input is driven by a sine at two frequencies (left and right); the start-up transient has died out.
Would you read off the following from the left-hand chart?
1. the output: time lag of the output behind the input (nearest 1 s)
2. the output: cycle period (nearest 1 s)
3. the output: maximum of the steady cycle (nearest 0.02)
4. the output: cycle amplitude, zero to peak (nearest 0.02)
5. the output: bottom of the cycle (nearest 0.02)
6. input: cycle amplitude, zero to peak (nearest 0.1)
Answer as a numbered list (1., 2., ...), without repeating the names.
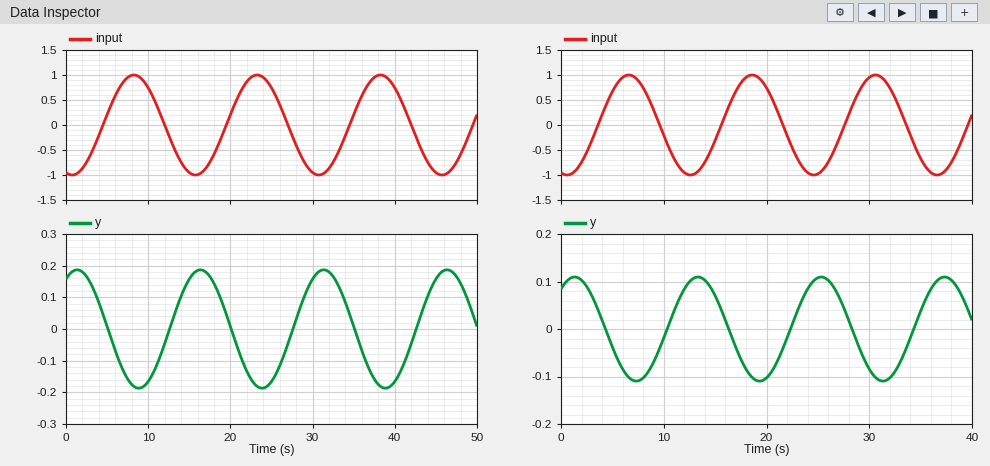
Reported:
1. 8 s
2. 15 s
3. 0.18
4. 0.18
5. -0.18
6. 1.0
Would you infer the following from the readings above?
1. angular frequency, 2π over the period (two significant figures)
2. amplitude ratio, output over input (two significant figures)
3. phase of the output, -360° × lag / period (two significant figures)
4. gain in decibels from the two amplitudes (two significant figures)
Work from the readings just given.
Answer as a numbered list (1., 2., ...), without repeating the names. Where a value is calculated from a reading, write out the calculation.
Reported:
1. 2π / 15 = 0.42 rad/s
2. 0.18 / 1 = 0.18
3. -360 × 8 / 15 = -190°
4. 20 log10(0.18 / 1) = -15 dB
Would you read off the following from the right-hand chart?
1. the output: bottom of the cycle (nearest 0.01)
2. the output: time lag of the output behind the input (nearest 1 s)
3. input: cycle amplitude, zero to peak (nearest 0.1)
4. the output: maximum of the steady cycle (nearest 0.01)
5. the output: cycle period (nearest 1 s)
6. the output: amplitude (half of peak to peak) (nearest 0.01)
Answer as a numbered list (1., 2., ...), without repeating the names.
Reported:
1. -0.11
2. 7 s
3. 1.0
4. 0.11
5. 12 s
6. 0.11
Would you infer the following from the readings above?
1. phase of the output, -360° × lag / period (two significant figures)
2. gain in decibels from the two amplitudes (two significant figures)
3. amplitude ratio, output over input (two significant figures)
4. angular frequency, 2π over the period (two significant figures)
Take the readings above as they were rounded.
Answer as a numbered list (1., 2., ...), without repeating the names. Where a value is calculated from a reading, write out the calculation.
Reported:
1. -360 × 7 / 12 = -210°
2. 20 log10(0.11 / 1) = -19 dB
3. 0.11 / 1 = 0.11
4. 2π / 12 = 0.52 rad/s
